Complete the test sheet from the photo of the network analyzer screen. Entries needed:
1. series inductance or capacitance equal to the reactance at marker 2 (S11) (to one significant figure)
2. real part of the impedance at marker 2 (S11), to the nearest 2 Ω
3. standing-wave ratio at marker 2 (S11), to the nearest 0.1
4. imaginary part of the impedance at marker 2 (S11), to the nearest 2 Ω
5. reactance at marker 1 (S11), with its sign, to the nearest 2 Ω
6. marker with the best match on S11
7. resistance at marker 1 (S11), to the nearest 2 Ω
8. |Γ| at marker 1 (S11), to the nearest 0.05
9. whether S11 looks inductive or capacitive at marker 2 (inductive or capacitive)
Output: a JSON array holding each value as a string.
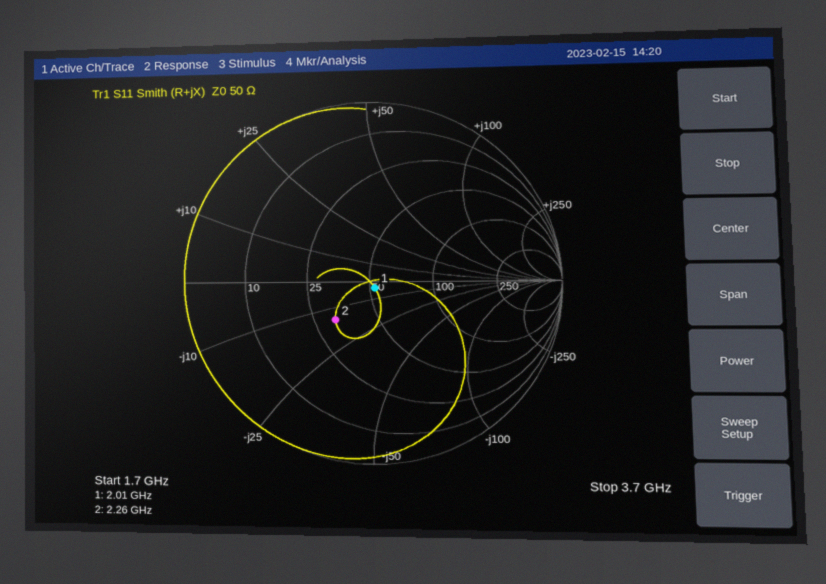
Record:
["5 pF", "32 Ω", "1.8", "-14 Ω", "-4 Ω", "marker 1", "52 Ω", "0.05", "capacitive"]
